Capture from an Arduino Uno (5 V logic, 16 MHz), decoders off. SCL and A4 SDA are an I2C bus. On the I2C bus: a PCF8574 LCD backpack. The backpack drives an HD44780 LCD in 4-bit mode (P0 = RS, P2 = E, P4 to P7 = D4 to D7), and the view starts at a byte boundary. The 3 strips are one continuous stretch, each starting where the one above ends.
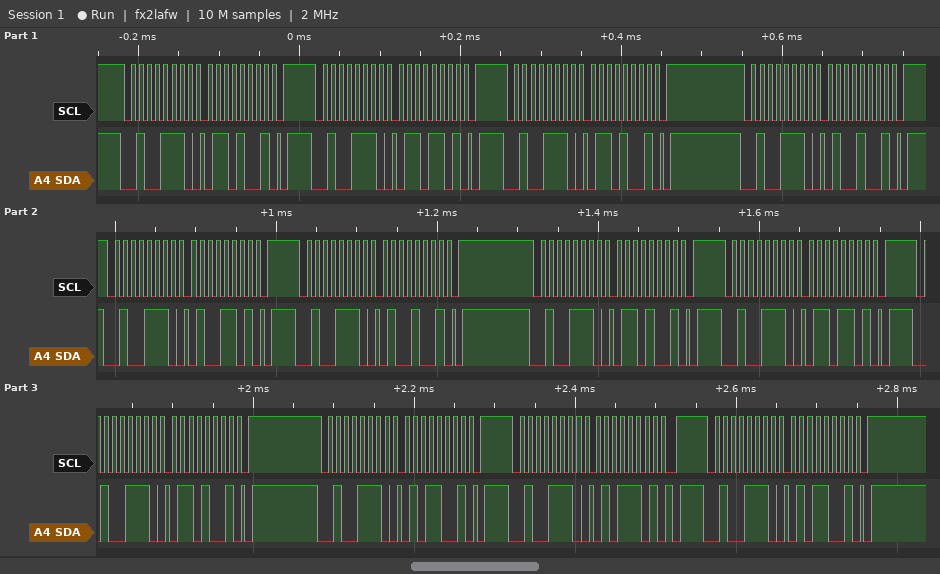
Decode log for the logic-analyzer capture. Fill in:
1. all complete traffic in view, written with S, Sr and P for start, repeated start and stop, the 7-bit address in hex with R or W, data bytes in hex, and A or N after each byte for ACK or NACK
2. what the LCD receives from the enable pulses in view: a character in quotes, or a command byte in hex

S 27W A 69 A P S 27W A 6D A P S 27W A 69 A P S 27W A 49 A P S 27W A 4D A P S 27W A 49 A P S 27W A 69 A P S 27W A 6D A P S 27W A 69 A P S 27W A 59 A P S 27W A 5D A P S 27W A 59 A P
'd' 'e'
